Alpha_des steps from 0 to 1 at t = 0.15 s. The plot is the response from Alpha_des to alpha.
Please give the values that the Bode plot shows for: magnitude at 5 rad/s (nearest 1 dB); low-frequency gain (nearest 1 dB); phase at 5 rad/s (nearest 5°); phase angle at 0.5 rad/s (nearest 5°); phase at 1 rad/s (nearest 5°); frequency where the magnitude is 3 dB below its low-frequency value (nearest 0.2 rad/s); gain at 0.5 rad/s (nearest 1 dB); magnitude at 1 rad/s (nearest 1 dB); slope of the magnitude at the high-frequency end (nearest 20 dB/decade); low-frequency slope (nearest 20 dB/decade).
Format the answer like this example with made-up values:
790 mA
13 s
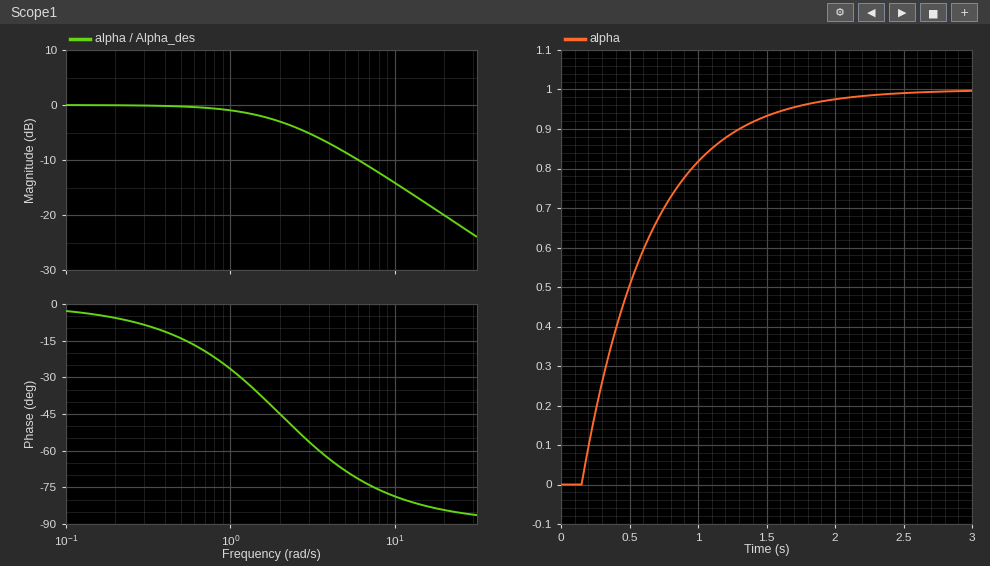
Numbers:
-9 dB
0 dB
-70°
-15°
-25°
2.0 rad/s
0 dB
-1 dB
-20 dB/decade
0 dB/decade
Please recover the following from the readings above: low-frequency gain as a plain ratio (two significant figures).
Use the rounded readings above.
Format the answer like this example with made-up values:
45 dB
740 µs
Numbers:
1.0
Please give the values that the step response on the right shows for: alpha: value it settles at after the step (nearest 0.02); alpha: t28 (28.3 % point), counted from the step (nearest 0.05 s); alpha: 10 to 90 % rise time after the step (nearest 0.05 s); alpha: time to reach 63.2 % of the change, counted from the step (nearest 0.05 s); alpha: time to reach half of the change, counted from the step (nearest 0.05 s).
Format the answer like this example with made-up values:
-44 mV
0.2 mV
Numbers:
1.00
0.15 s
1.10 s
0.50 s
0.35 s
